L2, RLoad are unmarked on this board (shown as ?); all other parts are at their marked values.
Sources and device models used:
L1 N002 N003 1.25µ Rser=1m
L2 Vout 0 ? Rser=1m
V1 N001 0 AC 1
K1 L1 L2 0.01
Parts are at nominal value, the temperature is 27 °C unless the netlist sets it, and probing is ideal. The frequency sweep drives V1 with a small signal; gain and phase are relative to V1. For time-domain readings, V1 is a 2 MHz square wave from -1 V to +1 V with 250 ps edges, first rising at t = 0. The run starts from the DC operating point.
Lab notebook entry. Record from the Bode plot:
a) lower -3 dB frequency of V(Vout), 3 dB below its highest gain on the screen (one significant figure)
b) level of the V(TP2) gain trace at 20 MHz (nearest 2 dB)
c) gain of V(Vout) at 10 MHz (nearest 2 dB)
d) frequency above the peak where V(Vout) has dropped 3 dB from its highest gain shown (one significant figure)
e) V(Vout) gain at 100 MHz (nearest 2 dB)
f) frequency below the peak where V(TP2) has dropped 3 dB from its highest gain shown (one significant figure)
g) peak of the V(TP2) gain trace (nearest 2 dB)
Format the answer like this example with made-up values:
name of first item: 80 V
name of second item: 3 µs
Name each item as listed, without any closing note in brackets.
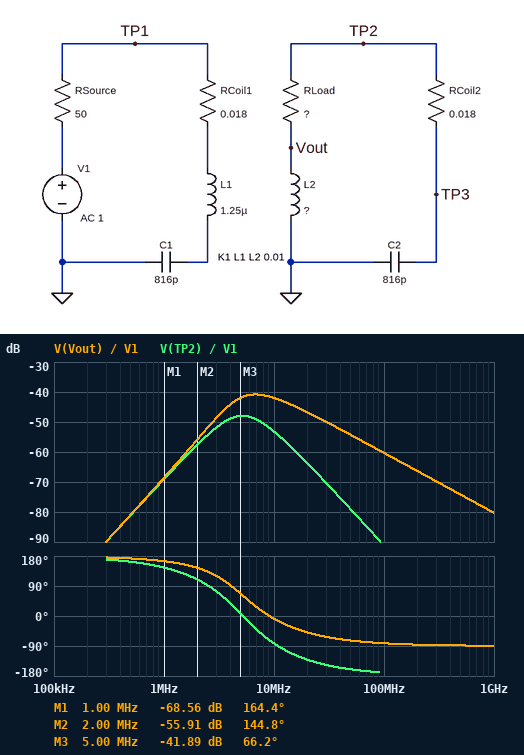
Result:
lower -3 dB frequency of V(Vout), 3 dB below its highest gain on the screen: 4 MHz
level of the V(TP2) gain trace at 20 MHz: -64 dB
gain of V(Vout) at 10 MHz: -42 dB
frequency above the peak where V(Vout) has dropped 3 dB from its highest gain shown: 10 MHz
V(Vout) gain at 100 MHz: -60 dB
frequency below the peak where V(TP2) has dropped 3 dB from its highest gain shown: 3 MHz
peak of the V(TP2) gain trace: -48 dB
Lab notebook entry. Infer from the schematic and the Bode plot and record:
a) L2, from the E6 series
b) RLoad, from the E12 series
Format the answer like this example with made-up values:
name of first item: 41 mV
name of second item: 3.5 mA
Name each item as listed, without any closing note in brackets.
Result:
L2, from the E6 series: 1 µH
RLoad, from the E12 series: 68 Ω
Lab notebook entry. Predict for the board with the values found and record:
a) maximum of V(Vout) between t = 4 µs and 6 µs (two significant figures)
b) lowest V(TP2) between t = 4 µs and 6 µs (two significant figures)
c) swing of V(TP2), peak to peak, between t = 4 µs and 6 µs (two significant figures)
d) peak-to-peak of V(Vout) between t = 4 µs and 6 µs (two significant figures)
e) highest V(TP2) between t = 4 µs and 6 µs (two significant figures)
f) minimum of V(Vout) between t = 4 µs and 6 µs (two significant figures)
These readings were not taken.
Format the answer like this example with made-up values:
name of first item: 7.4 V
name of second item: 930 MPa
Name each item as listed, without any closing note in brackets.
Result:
maximum of V(Vout) between t = 4 µs and 6 µs: 8.7 mV
lowest V(TP2) between t = 4 µs and 6 µs: -3.4 mV
swing of V(TP2), peak to peak, between t = 4 µs and 6 µs: 6.7 mV
peak-to-peak of V(Vout) between t = 4 µs and 6 µs: 17 mV
highest V(TP2) between t = 4 µs and 6 µs: 3.4 mV
minimum of V(Vout) between t = 4 µs and 6 µs: -8.7 mV
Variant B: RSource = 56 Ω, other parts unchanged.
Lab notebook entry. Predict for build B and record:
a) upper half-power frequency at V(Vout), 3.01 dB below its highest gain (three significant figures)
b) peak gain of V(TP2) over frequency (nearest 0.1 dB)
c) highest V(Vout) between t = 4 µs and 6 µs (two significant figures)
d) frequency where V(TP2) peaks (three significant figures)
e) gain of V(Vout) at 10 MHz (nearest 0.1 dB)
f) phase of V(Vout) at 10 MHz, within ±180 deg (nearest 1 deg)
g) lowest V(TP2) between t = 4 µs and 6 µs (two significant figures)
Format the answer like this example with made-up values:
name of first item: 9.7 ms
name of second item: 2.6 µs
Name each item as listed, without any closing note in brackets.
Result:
upper half-power frequency at V(Vout), 3.01 dB below its highest gain: 14.7 MHz
peak gain of V(TP2) over frequency: -48.9 dB
highest V(Vout) between t = 4 µs and 6 µs: 8.4 mV
frequency where V(TP2) peaks: 5.18 MHz
gain of V(Vout) at 10 MHz: -42.4 dB
phase of V(Vout) at 10 MHz, within ±180 deg: -5 deg
lowest V(TP2) between t = 4 µs and 6 µs: -3.2 mV
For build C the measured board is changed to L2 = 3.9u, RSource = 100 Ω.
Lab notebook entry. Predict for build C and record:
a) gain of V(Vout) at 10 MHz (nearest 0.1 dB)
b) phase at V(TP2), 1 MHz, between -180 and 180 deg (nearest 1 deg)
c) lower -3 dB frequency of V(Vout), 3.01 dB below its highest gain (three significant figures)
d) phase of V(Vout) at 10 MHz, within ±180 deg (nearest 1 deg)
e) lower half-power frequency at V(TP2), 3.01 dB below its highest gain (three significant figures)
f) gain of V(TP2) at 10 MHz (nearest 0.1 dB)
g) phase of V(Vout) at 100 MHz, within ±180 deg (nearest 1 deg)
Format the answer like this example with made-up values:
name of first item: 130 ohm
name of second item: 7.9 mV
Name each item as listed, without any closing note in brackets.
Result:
gain of V(Vout) at 10 MHz: -48.9 dB
phase at V(TP2), 1 MHz, between -180 and 180 deg: 130 deg
lower -3 dB frequency of V(Vout), 3.01 dB below its highest gain: 2.30 MHz
phase of V(Vout) at 10 MHz, within ±180 deg: -30 deg
lower half-power frequency at V(TP2), 3.01 dB below its highest gain: 2.04 MHz
gain of V(TP2) at 10 MHz: -60.1 dB
phase of V(Vout) at 100 MHz, within ±180 deg: -83 deg
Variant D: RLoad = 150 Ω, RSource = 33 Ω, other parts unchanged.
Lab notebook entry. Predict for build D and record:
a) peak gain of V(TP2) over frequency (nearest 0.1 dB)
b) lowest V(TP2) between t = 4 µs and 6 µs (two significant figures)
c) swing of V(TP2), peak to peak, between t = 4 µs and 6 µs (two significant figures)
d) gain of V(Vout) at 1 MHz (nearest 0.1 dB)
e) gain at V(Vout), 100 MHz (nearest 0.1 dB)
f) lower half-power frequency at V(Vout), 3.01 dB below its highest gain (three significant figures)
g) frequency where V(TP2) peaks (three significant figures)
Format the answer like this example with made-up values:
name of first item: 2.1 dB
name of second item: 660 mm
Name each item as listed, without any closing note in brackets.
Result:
peak gain of V(TP2) over frequency: -51.2 dB
lowest V(TP2) between t = 4 µs and 6 µs: -2.3 mV
swing of V(TP2), peak to peak, between t = 4 µs and 6 µs: 4.6 mV
gain of V(Vout) at 1 MHz: -68.5 dB
gain at V(Vout), 100 MHz: -53.6 dB
lower half-power frequency at V(Vout), 3.01 dB below its highest gain: 4.16 MHz
frequency where V(TP2) peaks: 5.00 MHz
